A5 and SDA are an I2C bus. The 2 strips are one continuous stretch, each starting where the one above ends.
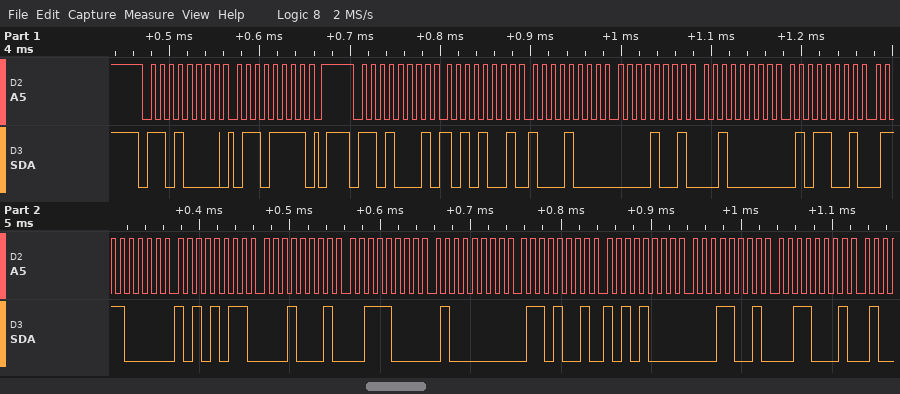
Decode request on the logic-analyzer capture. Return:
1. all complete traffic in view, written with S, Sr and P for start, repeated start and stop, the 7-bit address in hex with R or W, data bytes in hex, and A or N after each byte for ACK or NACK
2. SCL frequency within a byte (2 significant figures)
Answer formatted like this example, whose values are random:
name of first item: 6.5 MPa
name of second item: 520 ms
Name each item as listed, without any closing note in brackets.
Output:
all complete traffic in view, written with S, Sr and P for start, repeated start and stop, the 7-bit address in hex with R or W, data bytes in hex, and A or N after each byte for ACK or NACK: S 68W A 6F A P S 68R A A9 A 88 A 09 A 20 A 59 A 70 A AB A 11 A 38 A 40 A 69 A A8 A 19 A 31 A
SCL frequency within a byte: 100 kHz
